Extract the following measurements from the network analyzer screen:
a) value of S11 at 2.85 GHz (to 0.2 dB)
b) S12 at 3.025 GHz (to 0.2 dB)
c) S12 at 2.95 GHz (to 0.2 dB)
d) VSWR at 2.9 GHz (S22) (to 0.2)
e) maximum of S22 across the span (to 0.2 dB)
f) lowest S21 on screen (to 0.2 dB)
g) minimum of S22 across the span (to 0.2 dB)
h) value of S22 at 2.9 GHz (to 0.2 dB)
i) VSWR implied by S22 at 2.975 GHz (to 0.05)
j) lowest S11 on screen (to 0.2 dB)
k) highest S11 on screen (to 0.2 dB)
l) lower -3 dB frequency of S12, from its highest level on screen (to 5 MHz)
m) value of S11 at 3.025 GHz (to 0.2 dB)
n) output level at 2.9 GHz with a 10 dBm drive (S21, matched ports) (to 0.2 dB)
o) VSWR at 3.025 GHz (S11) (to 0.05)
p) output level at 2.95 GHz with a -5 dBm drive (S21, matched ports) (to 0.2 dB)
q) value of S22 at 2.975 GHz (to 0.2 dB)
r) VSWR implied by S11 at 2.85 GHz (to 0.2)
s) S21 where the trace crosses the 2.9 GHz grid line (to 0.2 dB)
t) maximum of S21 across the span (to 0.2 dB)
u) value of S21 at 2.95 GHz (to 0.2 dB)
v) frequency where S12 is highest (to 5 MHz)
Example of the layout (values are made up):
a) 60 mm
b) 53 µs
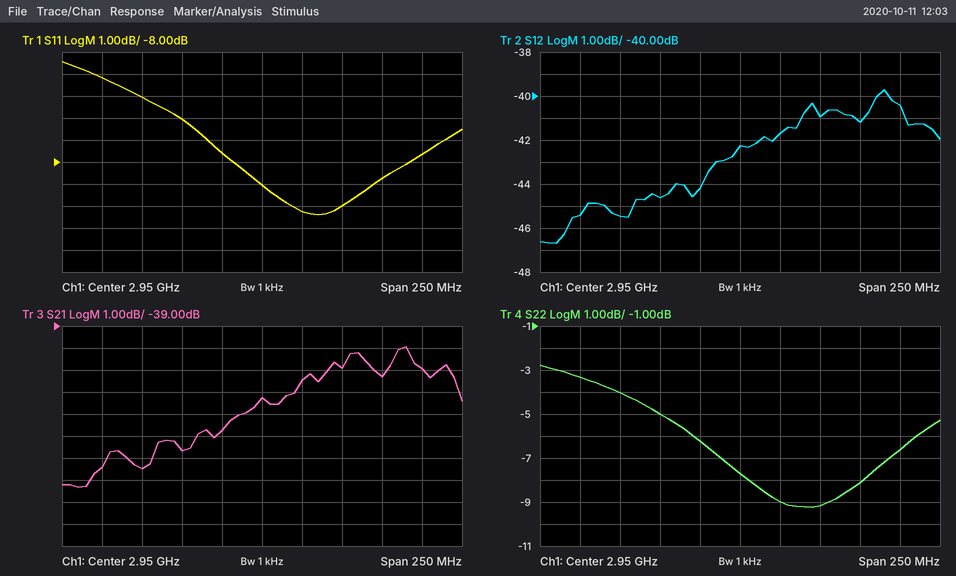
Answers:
a) -4.2 dB
b) -41.2 dB
c) -42.2 dB
d) 3.6
e) -2.8 dB
f) -46.4 dB
g) -9.2 dB
h) -5.0 dB
i) 2.10
j) -10.4 dB
k) -3.4 dB
l) 2.945 GHz
m) -8.8 dB
n) -34.6 dBm
o) 2.15
p) -47.2 dBm
q) -9.0 dB
r) 4.2
s) -44.6 dB
t) -40.0 dB
u) -42.2 dB
v) 3.040 GHz
